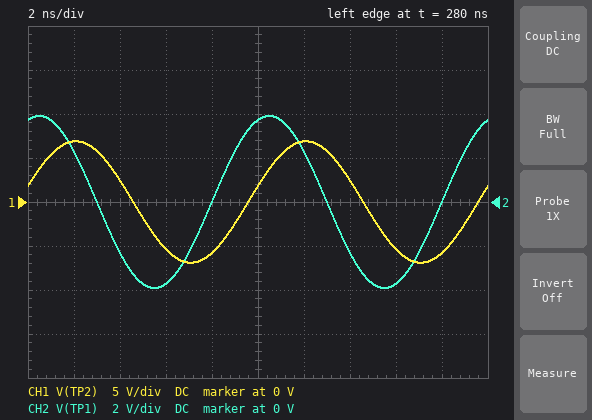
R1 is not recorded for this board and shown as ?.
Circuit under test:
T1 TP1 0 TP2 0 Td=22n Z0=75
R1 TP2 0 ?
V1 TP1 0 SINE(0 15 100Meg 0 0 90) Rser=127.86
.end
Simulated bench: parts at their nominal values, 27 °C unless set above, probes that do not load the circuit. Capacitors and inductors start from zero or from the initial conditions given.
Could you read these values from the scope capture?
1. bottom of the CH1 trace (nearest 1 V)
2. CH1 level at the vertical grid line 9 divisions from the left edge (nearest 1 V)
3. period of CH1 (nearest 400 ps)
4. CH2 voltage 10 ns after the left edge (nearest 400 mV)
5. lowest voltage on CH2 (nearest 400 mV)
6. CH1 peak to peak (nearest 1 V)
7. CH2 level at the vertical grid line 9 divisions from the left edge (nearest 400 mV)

-7 V
-6 V
10.0 ns
3.6 V
-4.0 V
14 V
0 V
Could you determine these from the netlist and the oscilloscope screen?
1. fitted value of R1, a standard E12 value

150 Ω
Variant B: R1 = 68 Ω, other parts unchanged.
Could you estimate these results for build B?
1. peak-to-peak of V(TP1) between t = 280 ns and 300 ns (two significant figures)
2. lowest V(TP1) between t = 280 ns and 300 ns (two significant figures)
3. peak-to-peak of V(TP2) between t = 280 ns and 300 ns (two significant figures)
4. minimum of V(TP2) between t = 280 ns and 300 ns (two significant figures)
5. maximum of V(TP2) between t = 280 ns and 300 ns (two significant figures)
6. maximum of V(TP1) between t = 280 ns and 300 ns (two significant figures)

12 V
-5.8 V
11 V
-5.3 V
5.3 V
5.8 V
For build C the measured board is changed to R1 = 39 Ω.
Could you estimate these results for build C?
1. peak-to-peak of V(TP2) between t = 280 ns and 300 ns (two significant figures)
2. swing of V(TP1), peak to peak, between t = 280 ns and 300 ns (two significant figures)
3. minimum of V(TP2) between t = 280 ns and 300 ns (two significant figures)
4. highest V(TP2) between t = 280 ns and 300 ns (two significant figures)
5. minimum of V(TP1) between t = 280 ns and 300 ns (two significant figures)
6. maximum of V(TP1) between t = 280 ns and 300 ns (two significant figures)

8.1 V
15 V
-4.1 V
4.1 V
-7.5 V
7.5 V
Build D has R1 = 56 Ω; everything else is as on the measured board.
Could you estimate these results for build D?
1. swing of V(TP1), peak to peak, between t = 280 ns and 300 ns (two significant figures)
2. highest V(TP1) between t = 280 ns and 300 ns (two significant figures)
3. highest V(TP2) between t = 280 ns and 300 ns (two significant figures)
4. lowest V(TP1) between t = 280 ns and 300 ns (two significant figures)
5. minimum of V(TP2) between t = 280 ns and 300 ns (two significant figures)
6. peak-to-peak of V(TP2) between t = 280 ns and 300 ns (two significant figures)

13 V
6.4 V
4.9 V
-6.4 V
-4.9 V
9.8 V
